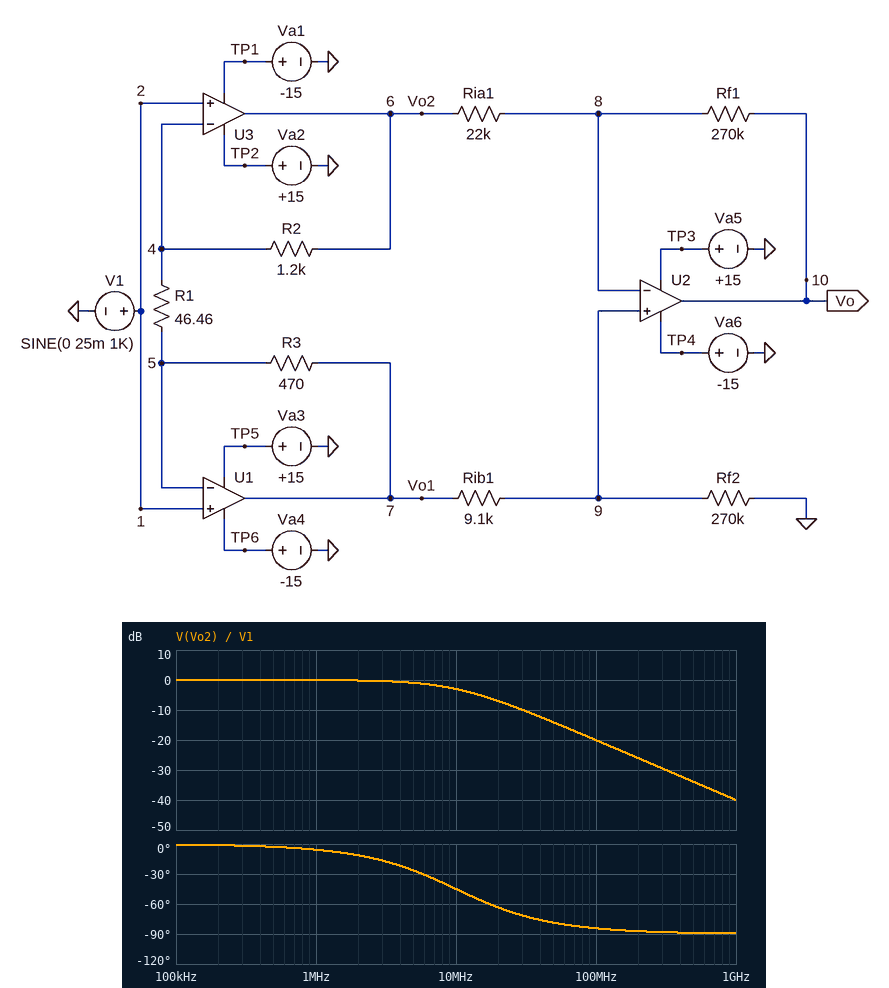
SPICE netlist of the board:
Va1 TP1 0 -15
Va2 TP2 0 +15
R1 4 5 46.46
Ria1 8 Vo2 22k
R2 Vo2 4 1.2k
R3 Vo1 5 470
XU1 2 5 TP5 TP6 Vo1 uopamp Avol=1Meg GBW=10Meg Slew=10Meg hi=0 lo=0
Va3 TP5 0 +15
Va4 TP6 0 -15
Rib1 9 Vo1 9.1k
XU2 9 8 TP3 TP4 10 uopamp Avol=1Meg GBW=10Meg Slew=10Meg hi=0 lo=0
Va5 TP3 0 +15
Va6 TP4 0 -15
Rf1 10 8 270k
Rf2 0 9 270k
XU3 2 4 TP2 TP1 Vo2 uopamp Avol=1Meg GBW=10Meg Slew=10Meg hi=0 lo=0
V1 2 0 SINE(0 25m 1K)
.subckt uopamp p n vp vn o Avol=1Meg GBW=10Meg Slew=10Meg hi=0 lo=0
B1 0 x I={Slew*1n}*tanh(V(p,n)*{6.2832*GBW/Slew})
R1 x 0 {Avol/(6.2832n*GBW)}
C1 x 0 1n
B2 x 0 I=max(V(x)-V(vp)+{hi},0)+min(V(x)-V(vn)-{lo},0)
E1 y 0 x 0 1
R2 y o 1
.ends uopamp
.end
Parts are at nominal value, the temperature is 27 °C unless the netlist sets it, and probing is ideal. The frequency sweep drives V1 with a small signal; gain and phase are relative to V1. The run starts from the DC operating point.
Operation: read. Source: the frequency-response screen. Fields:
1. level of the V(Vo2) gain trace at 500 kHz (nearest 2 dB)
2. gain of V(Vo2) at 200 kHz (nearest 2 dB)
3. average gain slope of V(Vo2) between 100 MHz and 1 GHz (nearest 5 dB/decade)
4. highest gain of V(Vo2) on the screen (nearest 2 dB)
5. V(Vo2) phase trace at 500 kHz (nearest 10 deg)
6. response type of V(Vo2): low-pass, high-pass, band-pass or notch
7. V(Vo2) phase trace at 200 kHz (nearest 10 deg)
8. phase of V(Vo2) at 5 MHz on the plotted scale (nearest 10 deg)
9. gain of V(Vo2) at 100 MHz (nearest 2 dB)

0 dB
0 dB
-20 dB/decade
0 dB
0 deg
low-pass
0 deg
-30 deg
-20 dB
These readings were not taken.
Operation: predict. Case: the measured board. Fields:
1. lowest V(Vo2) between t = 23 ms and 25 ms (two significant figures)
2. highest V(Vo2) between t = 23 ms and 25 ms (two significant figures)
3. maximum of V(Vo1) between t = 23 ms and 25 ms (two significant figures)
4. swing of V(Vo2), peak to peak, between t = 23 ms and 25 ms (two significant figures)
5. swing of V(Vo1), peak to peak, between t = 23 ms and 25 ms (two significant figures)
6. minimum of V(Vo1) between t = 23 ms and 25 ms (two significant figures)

-25 mV
25 mV
25 mV
50 mV
50 mV
-25 mV
